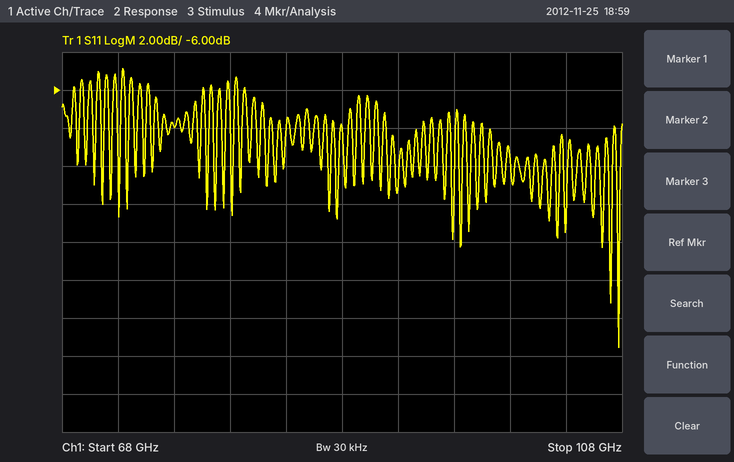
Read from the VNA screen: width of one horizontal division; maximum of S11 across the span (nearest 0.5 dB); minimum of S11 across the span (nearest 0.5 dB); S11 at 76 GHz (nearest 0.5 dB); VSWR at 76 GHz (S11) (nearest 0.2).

4 GHz
-5.0 dB
-19.5 dB
-8.0 dB
2.4
